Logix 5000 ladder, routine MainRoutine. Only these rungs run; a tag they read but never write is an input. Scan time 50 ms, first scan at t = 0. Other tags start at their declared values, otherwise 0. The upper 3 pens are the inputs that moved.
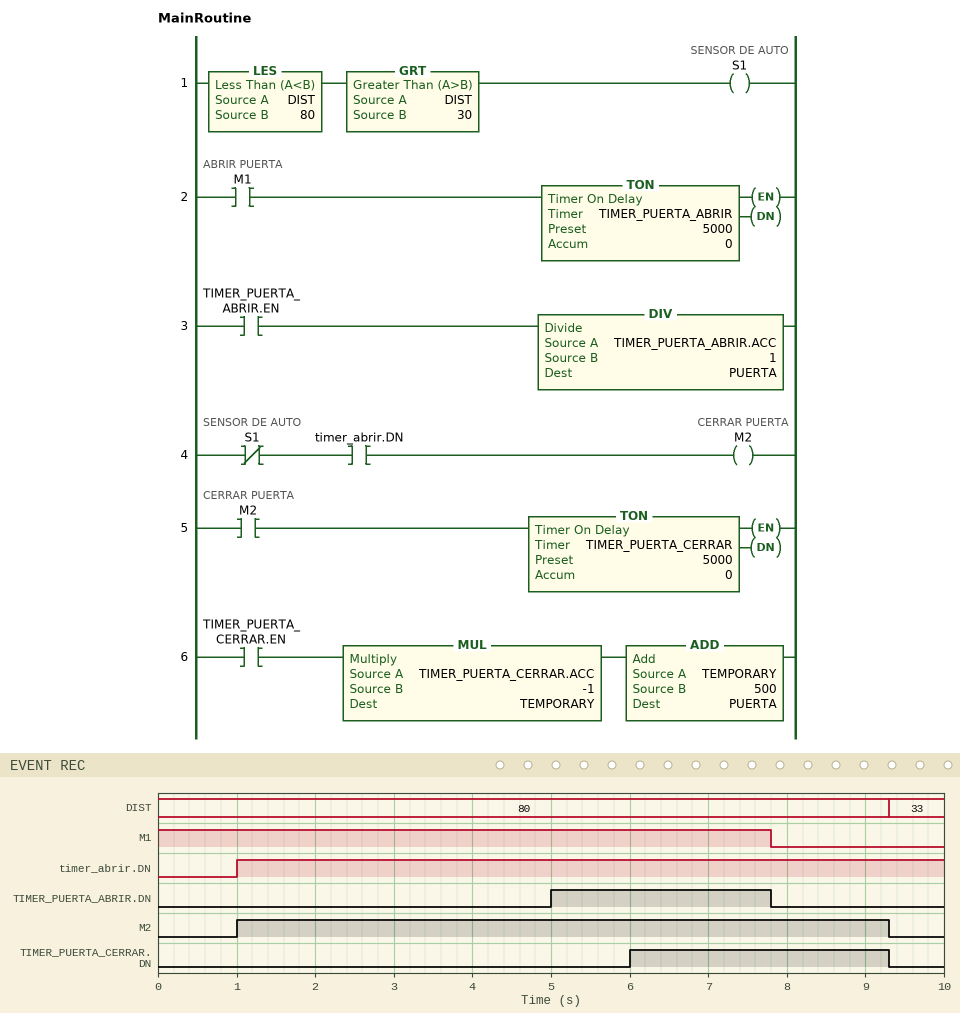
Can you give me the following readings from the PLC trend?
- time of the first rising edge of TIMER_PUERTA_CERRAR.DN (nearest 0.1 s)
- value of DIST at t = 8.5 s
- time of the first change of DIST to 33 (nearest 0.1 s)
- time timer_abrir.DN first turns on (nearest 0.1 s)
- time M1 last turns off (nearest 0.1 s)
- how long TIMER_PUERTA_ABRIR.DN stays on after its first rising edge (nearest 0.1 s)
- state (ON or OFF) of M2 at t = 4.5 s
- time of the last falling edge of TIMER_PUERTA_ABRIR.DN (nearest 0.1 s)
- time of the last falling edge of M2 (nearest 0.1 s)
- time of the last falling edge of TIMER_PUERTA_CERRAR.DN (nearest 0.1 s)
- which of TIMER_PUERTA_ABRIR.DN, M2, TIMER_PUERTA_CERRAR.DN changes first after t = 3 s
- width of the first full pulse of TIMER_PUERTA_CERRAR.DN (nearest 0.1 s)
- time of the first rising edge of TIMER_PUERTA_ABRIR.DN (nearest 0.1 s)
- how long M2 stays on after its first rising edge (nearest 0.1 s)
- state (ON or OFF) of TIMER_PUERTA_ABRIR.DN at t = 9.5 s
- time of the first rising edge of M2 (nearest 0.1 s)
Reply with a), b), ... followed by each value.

a) 6.0 s
b) 80
c) 9.3 s
d) 1.0 s
e) 7.8 s
f) 2.8 s
g) ON
h) 7.8 s
i) 9.3 s
j) 9.3 s
k) TIMER_PUERTA_ABRIR.DN
l) 3.3 s
m) 5.0 s
n) 8.3 s
o) OFF
p) 1.0 s
